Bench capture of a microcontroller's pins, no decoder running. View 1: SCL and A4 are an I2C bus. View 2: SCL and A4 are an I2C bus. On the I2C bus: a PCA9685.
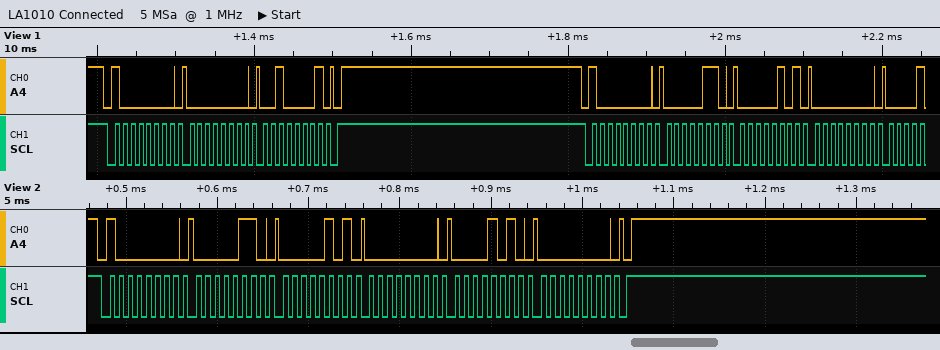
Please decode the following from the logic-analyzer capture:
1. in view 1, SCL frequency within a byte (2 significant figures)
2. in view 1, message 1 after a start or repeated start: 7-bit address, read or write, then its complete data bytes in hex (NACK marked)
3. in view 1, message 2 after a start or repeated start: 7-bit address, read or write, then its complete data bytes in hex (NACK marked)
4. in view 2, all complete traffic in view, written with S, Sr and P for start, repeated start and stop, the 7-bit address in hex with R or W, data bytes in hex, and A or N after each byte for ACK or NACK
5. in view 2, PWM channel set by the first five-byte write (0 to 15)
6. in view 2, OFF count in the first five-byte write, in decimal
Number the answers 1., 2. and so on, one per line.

1. 100 kHz
2. 0x40 write: 00 21
3. 0x40 write: 06 05 00
4. S 40W A 06 A 05 A 00 A 0A A 00 A P
5. 0
6. 10
